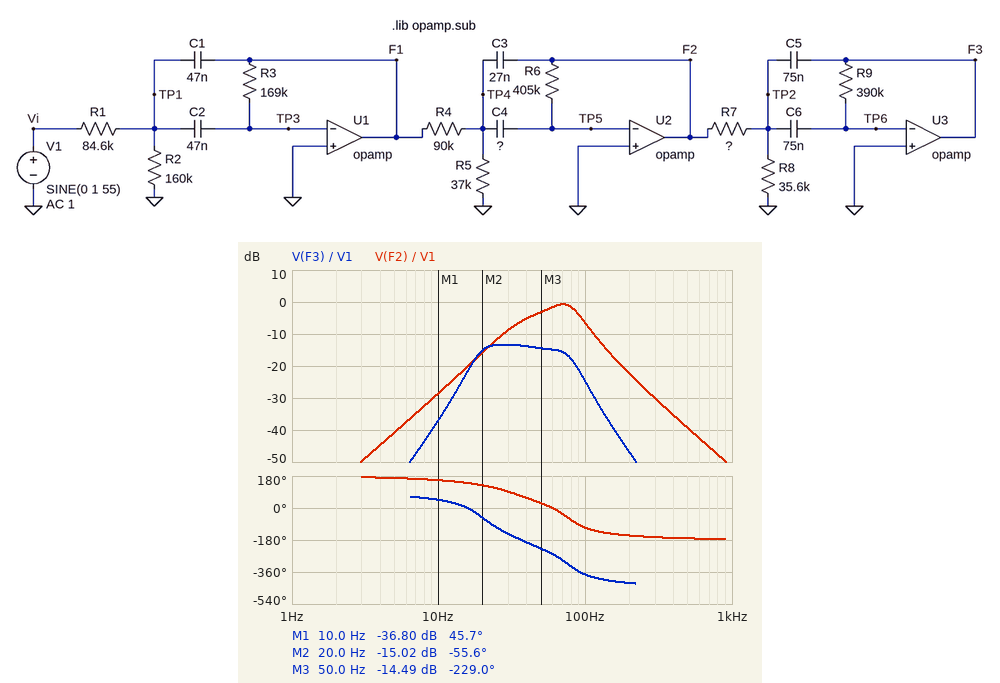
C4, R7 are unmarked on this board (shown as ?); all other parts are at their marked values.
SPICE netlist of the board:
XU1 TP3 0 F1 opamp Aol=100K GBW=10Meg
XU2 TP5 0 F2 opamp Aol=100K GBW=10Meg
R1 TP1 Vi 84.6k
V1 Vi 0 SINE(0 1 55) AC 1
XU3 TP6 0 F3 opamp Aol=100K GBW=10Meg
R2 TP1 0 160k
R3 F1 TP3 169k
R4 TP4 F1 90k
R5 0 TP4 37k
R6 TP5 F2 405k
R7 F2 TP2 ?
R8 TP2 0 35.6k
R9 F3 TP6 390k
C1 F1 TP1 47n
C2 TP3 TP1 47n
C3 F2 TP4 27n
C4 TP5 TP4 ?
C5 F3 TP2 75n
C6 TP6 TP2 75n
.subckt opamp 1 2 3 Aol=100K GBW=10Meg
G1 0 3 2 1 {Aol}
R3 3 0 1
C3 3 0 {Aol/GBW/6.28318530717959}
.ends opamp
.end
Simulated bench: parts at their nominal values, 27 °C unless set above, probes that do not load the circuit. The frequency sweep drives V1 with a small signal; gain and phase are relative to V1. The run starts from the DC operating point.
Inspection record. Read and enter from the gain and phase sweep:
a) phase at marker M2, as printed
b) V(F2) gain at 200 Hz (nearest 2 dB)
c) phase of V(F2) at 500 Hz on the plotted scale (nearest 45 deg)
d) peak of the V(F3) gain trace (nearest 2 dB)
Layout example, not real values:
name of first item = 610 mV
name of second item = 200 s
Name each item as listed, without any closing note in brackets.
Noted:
phase at marker M2, as printed = -55.6 deg
V(F2) gain at 200 Hz = -22 dB
phase of V(F2) at 500 Hz on the plotted scale = -180 deg
peak of the V(F3) gain trace = -14 dB
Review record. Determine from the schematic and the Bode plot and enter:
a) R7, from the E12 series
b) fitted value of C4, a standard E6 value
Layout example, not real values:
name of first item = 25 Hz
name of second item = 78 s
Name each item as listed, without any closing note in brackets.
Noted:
R7, from the E12 series = 180 kΩ
fitted value of C4, a standard E6 value = 15 nF
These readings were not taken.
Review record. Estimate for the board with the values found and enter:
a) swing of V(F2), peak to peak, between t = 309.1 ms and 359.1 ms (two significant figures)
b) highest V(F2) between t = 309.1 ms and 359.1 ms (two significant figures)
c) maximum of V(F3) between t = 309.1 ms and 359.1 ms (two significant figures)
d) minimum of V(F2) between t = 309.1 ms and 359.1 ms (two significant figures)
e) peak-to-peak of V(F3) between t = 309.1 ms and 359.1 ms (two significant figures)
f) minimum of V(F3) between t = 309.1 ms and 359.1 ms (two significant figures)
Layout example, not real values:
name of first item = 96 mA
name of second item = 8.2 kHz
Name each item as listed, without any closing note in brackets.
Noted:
swing of V(F2), peak to peak, between t = 309.1 ms and 359.1 ms = 1.5 V
highest V(F2) between t = 309.1 ms and 359.1 ms = 770 mV
maximum of V(F3) between t = 309.1 ms and 359.1 ms = 180 mV
minimum of V(F2) between t = 309.1 ms and 359.1 ms = -770 mV
peak-to-peak of V(F3) between t = 309.1 ms and 359.1 ms = 370 mV
minimum of V(F3) between t = 309.1 ms and 359.1 ms = -180 mV
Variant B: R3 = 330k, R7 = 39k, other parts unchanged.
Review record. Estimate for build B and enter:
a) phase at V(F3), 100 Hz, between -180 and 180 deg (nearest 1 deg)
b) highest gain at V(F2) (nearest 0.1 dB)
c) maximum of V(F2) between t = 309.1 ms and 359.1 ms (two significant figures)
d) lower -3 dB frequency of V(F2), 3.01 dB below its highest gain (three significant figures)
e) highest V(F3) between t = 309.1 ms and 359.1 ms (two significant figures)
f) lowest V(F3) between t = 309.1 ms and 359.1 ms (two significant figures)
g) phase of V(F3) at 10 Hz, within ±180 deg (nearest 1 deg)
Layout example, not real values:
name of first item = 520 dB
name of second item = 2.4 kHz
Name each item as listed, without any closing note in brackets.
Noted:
phase at V(F3), 100 Hz, between -180 and 180 deg = -26 deg
highest gain at V(F2) = -0.5 dB
maximum of V(F2) between t = 309.1 ms and 359.1 ms = 820 mV
lower -3 dB frequency of V(F2), 3.01 dB below its highest gain = 28.6 Hz
highest V(F3) between t = 309.1 ms and 359.1 ms = 990 mV
lowest V(F3) between t = 309.1 ms and 359.1 ms = -990 mV
phase of V(F3) at 10 Hz, within ±180 deg = 53 deg
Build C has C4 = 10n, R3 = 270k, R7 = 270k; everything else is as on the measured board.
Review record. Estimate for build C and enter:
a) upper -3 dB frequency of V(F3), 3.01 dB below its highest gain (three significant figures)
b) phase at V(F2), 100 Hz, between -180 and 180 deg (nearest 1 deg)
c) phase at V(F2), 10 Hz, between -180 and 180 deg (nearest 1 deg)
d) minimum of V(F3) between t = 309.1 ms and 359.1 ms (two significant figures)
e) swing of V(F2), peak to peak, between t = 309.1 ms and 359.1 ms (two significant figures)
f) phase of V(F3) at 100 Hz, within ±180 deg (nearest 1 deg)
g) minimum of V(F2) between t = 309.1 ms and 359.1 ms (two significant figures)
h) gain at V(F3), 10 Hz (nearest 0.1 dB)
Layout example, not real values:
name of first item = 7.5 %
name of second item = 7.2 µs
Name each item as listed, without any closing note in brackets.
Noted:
upper -3 dB frequency of V(F3), 3.01 dB below its highest gain = 36.8 Hz
phase at V(F2), 100 Hz, between -180 and 180 deg = -87 deg
phase at V(F2), 10 Hz, between -180 and 180 deg = 156 deg
minimum of V(F3) between t = 309.1 ms and 359.1 ms = -73 mV
swing of V(F2), peak to peak, between t = 309.1 ms and 359.1 ms = 920 mV
phase of V(F3) at 100 Hz, within ±180 deg = 9 deg
minimum of V(F2) between t = 309.1 ms and 359.1 ms = -460 mV
gain at V(F3), 10 Hz = -38.8 dB
